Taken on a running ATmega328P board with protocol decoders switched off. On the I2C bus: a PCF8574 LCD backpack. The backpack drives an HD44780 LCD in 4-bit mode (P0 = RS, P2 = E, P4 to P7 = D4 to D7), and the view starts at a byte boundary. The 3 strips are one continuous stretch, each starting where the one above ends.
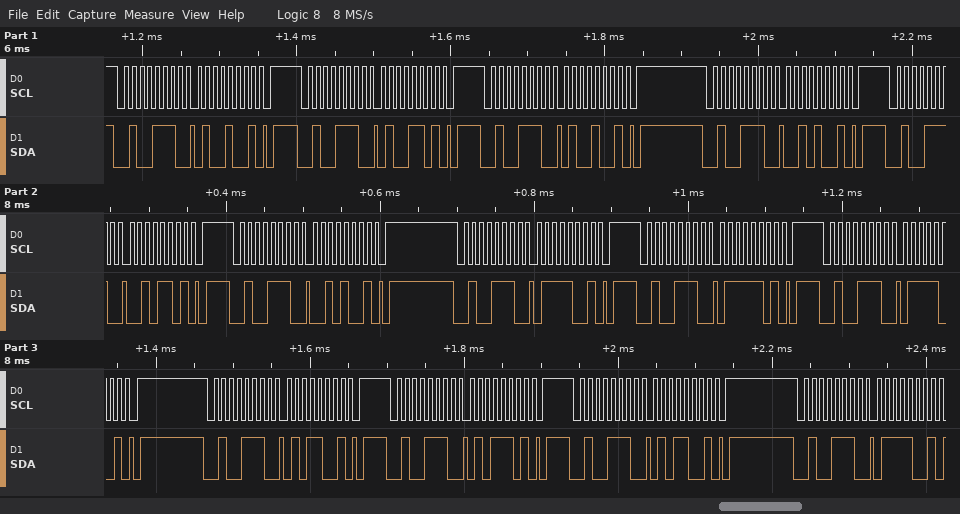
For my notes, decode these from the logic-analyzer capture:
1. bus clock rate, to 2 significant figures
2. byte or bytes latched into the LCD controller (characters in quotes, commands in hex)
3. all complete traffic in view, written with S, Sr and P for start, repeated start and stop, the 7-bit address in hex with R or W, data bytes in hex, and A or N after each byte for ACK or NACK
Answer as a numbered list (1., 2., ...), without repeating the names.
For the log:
1. 100 kHz
2. 'B' 'u'
3. S 27W A 49 A P S 27W A 4D A P S 27W A 49 A P S 27W A 29 A P S 27W A 2D A P S 27W A 29 A P S 27W A 79 A P S 27W A 7D A P S 27W A 79 A P S 27W A 59 A P S 27W A 5D A P S 27W A 59 A P S 27W A 79 A
